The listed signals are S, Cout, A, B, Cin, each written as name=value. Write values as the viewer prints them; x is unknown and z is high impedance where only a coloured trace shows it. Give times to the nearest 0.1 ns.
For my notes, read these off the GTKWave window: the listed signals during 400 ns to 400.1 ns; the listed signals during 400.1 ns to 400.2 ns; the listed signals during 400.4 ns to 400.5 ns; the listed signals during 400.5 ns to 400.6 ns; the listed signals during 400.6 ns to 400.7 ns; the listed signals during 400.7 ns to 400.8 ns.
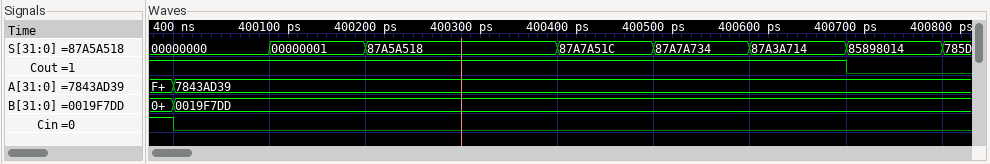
S=00000000, Cout=1, A=7843AD39, B=0019F7DD, Cin=0
S=00000001, Cout=1, A=7843AD39, B=0019F7DD, Cin=0
S=87A7A51C, Cout=1, A=7843AD39, B=0019F7DD, Cin=0
S=87A7A734, Cout=1, A=7843AD39, B=0019F7DD, Cin=0
S=87A3A714, Cout=1, A=7843AD39, B=0019F7DD, Cin=0
S=85898014, Cout=0, A=7843AD39, B=0019F7DD, Cin=0
